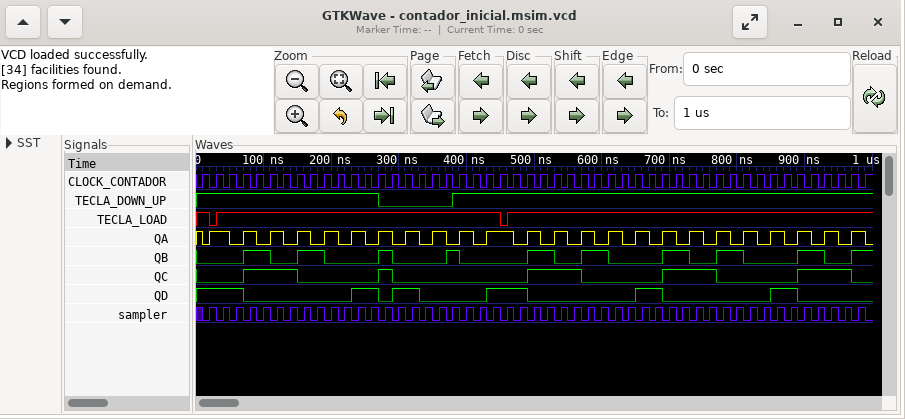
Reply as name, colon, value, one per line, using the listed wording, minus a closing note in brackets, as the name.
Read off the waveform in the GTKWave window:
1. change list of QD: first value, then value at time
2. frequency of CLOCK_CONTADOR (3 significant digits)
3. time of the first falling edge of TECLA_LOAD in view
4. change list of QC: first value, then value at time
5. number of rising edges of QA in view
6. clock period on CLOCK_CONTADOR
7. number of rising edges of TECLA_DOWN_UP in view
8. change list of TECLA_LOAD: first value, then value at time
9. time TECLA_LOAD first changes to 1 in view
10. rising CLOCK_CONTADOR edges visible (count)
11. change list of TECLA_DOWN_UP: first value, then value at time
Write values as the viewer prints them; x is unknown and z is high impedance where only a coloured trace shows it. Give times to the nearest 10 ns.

change list of QD: first value, then value at time: 1, 0 at 70 ns, 1 at 230 ns, 0 at 270 ns, 1 at 290 ns, 0 at 330 ns, 1 at 430 ns, 0 at 490 ns, 1 at 650 ns, 0 at 690 ns, 1 at 850 ns, 0 at 890 ns
frequency of CLOCK_CONTADOR: 50.0 MHz
time of the first falling edge of TECLA_LOAD in view: 20 ns
change list of QC: first value, then value at time: 0, 1 at 70 ns, 0 at 150 ns, 1 at 270 ns, 0 at 290 ns, 1 at 490 ns, 0 at 570 ns, 1 at 690 ns, 0 at 770 ns, 1 at 890 ns, 0 at 970 ns
number of rising edges of QA in view: 24
clock period on CLOCK_CONTADOR: 20 ns
number of rising edges of TECLA_DOWN_UP in view: 1
change list of TECLA_LOAD: first value, then value at time: 1, 0 at 20 ns, 1 at 30 ns, 0 at 450 ns, 1 at 460 ns
time TECLA_LOAD first changes to 1 in view: 30 ns
rising CLOCK_CONTADOR edges visible: 50
change list of TECLA_DOWN_UP: first value, then value at time: 1, 0 at 270 ns, 1 at 380 ns
